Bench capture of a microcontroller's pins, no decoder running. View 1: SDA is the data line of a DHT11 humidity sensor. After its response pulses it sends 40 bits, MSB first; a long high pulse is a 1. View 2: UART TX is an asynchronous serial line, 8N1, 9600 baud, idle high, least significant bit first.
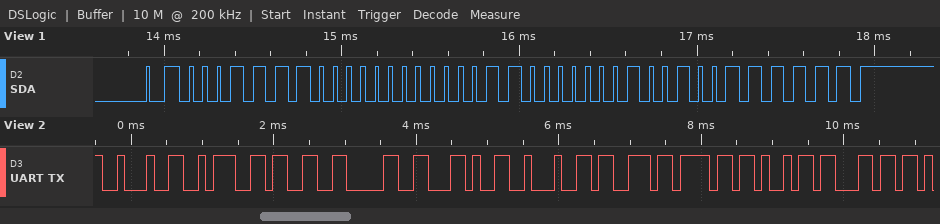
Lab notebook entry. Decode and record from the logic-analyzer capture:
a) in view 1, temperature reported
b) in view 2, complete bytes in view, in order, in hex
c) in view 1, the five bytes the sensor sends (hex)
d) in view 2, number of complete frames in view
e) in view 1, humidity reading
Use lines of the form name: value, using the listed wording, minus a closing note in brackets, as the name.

in view 1, temperature reported: 24.9 °C
in view 2, complete bytes in view, in order, in hex: 22 3A 33 30 2C 22 73 6F 69 6C
in view 1, the five bytes the sensor sends: 1E 00 18 09 3F
in view 2, number of complete frames in view: 10
in view 1, humidity reading: 30 %
